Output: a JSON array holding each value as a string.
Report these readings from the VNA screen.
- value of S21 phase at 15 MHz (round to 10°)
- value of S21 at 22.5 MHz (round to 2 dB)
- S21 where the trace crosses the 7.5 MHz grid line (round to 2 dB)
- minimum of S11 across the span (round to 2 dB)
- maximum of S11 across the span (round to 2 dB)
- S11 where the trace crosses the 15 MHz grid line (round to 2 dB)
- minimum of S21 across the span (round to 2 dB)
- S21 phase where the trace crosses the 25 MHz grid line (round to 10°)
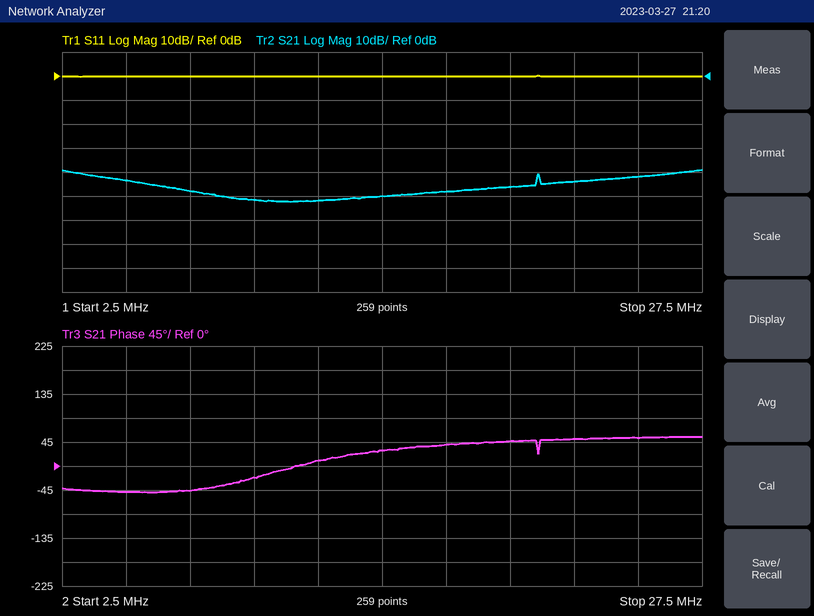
["30°", "-44 dB", "-48 dB", "0 dB", "0 dB", "0 dB", "-52 dB", "50°"]
